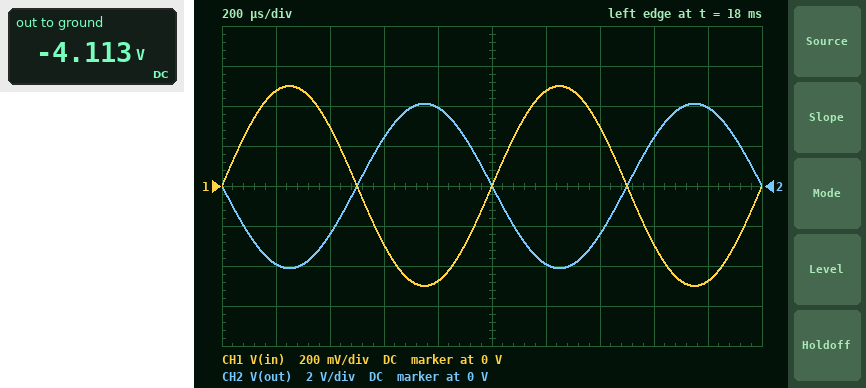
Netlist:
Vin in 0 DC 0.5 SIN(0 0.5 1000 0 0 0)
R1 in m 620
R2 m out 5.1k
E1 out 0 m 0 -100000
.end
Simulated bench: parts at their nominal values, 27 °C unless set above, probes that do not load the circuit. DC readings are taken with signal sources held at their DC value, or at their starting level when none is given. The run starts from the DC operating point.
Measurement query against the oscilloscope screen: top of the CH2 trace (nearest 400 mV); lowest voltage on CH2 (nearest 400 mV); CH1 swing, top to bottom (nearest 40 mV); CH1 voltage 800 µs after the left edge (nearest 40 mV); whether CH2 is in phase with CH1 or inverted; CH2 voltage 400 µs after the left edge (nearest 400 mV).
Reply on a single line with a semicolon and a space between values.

4.0 V; -4.0 V; 1.00 V; -480 mV; inverted; -2.4 V
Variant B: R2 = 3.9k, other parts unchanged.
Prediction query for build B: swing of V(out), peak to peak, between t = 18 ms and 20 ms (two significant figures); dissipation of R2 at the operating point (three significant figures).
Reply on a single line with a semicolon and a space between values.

6.3 V; 2.54 mW
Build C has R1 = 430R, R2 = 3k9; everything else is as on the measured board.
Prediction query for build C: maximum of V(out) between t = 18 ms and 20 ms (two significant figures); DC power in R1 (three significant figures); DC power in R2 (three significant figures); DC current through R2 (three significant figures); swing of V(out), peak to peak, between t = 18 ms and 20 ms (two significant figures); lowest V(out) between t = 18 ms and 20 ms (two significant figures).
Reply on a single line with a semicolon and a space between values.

4.5 V; 581 µW; 5.27 mW; 1.16 mA; 9.1 V; -4.5 V
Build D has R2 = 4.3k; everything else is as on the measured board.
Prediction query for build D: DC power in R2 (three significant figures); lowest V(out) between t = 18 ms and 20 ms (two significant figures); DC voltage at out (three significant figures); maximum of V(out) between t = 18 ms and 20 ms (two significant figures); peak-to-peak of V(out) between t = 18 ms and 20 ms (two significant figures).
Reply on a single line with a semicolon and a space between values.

2.80 mW; -3.5 V; -3.47 V; 3.5 V; 6.9 V
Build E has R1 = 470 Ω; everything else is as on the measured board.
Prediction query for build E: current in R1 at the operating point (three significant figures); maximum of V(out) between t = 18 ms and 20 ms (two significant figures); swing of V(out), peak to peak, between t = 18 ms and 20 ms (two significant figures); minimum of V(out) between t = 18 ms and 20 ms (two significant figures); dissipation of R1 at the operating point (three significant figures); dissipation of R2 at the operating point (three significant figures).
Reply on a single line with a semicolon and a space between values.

1.06 mA; 5.4 V; 11 V; -5.4 V; 532 µW; 5.77 mW
